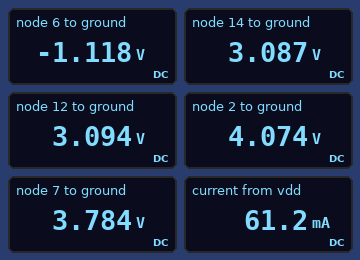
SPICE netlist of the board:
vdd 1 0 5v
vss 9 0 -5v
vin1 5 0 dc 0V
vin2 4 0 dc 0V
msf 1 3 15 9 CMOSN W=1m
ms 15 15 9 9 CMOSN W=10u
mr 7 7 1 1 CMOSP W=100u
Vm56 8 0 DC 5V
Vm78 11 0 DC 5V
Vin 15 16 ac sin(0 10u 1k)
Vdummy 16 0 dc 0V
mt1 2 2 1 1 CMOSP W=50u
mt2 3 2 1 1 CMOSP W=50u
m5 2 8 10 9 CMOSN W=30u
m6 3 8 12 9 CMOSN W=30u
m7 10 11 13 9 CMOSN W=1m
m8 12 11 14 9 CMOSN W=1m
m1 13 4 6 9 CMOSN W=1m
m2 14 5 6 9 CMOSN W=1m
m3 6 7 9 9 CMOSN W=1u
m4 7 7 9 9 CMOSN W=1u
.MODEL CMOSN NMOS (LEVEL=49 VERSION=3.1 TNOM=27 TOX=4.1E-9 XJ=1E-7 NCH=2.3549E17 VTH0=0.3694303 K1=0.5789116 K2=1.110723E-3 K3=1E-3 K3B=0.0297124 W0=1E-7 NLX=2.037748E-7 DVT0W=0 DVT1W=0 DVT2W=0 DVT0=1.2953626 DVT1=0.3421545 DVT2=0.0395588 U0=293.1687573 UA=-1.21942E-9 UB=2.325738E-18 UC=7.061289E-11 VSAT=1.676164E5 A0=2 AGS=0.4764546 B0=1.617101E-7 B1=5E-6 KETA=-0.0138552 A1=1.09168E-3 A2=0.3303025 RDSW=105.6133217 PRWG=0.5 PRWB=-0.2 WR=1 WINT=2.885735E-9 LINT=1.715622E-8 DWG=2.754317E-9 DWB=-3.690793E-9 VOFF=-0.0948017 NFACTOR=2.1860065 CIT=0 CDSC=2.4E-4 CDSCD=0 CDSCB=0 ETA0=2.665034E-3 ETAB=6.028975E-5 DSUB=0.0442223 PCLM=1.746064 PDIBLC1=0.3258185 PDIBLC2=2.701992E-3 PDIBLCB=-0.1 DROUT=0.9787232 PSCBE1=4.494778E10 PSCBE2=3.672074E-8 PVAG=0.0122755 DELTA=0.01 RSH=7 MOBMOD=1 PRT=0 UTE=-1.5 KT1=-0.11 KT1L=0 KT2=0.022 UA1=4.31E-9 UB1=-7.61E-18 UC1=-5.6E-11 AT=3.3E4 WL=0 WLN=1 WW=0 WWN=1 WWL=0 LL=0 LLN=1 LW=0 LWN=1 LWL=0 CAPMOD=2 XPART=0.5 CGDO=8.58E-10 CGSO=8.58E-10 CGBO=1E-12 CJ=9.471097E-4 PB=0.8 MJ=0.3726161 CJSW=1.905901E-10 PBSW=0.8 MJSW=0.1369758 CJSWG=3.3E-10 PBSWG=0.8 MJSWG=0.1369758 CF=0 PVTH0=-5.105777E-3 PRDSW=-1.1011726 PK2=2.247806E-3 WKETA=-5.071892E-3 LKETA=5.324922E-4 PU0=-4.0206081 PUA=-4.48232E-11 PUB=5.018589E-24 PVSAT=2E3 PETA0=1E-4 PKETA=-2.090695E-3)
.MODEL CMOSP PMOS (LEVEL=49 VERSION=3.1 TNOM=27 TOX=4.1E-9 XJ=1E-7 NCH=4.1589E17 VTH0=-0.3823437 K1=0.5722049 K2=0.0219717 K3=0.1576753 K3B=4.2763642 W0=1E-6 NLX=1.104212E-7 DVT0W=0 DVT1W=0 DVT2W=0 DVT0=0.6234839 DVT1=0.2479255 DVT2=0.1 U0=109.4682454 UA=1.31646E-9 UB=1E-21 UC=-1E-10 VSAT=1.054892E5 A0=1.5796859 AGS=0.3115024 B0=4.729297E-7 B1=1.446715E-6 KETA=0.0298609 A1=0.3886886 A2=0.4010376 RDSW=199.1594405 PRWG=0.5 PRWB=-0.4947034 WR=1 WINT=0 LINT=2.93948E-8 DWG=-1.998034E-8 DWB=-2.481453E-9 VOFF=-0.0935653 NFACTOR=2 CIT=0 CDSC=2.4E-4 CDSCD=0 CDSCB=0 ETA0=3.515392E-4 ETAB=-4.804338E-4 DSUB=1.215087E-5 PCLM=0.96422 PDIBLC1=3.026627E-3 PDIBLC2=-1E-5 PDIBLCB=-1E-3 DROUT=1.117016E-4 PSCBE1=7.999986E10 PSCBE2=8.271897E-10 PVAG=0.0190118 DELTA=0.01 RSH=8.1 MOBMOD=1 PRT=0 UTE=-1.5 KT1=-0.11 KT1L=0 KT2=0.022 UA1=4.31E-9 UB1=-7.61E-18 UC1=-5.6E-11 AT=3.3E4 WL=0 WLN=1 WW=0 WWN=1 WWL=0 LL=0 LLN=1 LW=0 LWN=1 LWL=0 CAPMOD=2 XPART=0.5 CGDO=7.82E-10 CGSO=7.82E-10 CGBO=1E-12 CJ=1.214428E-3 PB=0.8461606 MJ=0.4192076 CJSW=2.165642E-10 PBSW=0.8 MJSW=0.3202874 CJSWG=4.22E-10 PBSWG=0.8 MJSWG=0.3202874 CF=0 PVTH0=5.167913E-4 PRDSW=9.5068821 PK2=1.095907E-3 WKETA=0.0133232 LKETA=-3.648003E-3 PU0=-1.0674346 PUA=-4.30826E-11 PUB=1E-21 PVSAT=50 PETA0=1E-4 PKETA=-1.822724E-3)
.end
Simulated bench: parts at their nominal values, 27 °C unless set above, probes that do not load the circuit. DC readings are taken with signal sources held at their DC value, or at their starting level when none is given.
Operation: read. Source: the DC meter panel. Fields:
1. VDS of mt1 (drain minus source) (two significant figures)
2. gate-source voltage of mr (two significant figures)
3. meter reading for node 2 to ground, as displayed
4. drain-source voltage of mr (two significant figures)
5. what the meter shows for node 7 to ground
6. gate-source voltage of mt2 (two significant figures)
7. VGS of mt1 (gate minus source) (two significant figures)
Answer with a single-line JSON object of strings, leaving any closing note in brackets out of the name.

{"VDS of mt1 (drain minus source)": "-930 mV", "gate-source voltage of mr": "-1.2 V", "meter reading for node 2 to ground, as displayed": "4.074 V", "drain-source voltage of mr": "-1.2 V", "what the meter shows for node 7 to ground": "3.784 V", "gate-source voltage of mt2": "-930 mV", "VGS of mt1 (gate minus source)": "-930 mV"}
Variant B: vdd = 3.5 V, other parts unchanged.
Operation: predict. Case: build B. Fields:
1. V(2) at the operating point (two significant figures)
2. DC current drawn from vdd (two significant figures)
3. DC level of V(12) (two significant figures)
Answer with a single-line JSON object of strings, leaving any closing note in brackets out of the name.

{"V(2) at the operating point": "2.5 V", "DC current drawn from vdd": "22 mA", "DC level of V(12)": "2.4 V"}
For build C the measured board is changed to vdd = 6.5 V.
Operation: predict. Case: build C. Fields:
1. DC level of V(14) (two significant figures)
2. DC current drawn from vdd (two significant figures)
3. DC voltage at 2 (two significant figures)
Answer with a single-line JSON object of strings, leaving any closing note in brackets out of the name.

{"DC level of V(14)": "3.1 V", "DC current drawn from vdd": "99 mA", "DC voltage at 2": "5.6 V"}
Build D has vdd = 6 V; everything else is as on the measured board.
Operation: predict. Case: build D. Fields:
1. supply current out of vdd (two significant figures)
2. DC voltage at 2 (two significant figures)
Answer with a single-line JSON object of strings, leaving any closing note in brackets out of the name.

{"supply current out of vdd": "87 mA", "DC voltage at 2": "5.1 V"}
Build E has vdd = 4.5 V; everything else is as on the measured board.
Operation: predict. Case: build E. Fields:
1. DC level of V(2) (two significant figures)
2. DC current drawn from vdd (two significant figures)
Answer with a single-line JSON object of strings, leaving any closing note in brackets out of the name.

{"DC level of V(2)": "3.6 V", "DC current drawn from vdd": "48 mA"}
